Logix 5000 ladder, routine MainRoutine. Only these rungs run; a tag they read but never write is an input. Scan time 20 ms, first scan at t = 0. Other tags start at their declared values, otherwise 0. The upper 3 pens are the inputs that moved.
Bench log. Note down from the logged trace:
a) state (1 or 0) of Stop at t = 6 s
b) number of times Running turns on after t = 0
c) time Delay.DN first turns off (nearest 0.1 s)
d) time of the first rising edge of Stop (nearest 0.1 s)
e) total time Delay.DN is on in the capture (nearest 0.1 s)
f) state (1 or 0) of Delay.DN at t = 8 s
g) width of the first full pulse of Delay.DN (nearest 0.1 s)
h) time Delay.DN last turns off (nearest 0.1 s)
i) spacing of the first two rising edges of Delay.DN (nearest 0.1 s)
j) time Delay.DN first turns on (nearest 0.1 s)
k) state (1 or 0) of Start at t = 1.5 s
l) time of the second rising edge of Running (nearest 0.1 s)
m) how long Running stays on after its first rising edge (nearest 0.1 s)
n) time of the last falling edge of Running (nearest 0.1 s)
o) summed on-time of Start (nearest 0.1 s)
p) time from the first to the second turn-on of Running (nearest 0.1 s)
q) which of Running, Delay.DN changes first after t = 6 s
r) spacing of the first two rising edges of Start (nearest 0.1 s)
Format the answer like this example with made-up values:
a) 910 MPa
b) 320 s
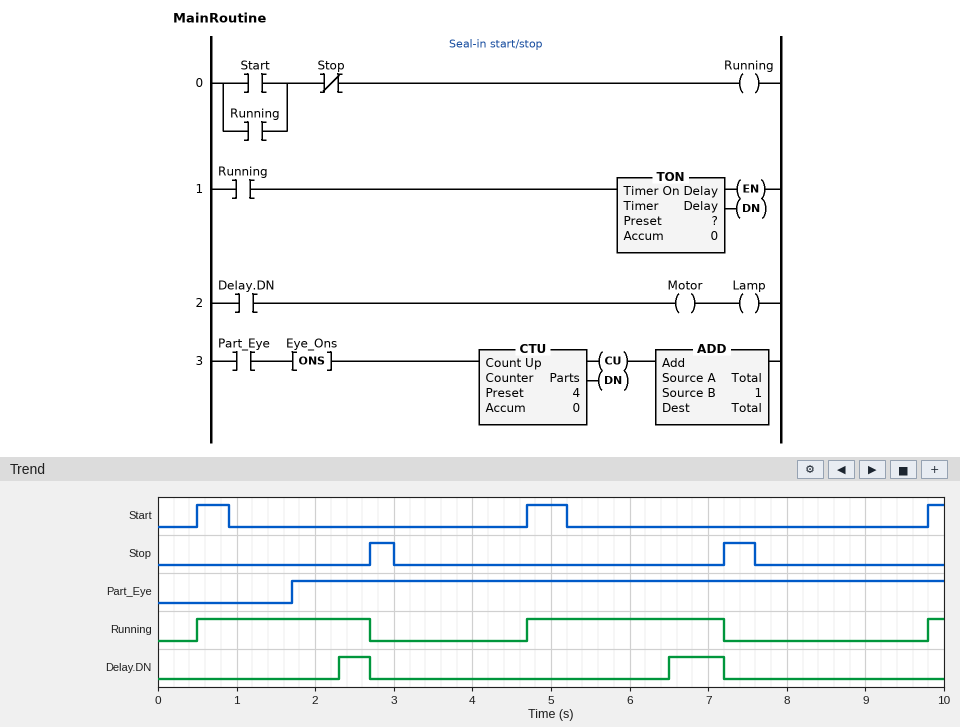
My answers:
a) 0
b) 3
c) 2.7 s
d) 2.7 s
e) 1.1 s
f) 0
g) 0.4 s
h) 7.2 s
i) 4.2 s
j) 2.3 s
k) 0
l) 4.7 s
m) 2.2 s
n) 7.2 s
o) 1.1 s
p) 4.2 s
q) Delay.DN
r) 4.2 s
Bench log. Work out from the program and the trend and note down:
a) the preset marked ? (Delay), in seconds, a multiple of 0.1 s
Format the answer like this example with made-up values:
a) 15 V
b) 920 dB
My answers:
a) 1.8 s
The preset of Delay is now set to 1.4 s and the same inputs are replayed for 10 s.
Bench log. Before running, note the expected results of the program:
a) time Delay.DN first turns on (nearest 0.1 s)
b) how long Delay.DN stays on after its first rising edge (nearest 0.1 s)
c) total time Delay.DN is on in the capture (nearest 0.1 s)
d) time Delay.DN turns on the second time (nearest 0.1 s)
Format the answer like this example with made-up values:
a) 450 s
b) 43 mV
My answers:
a) 1.9 s
b) 0.8 s
c) 1.9 s
d) 6.1 s
